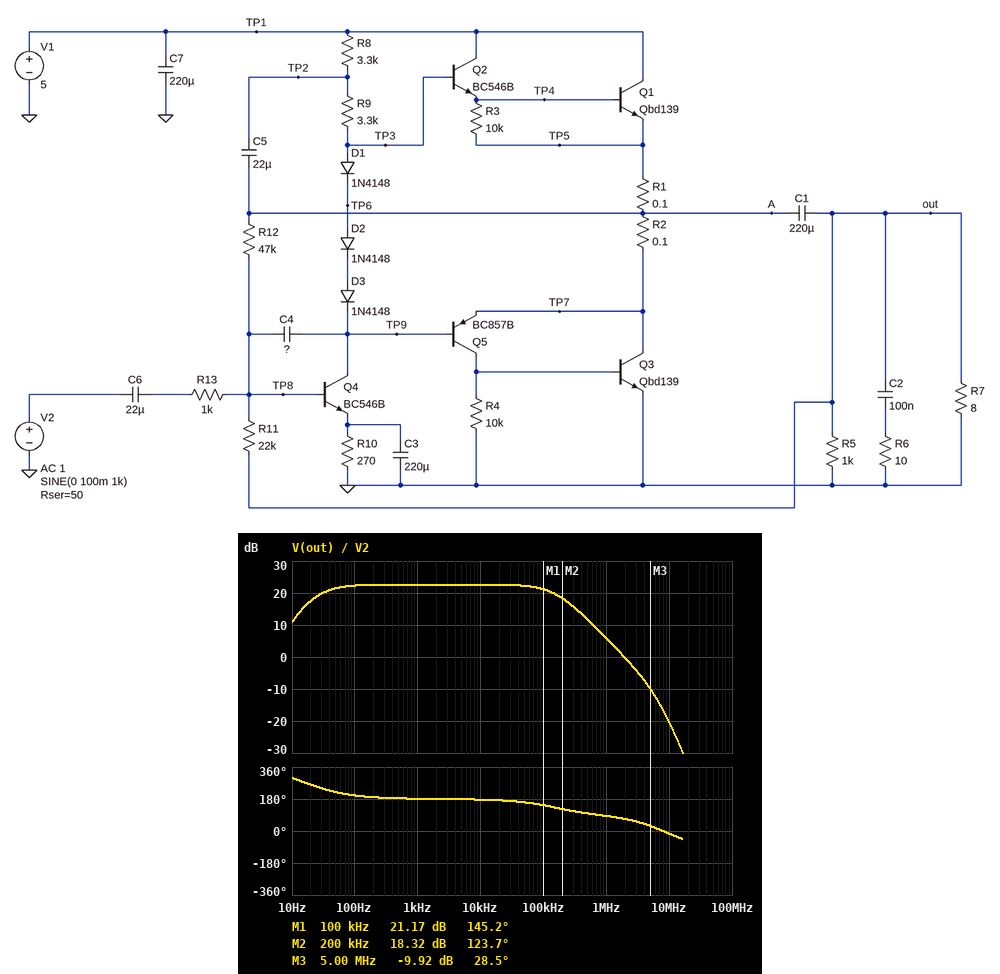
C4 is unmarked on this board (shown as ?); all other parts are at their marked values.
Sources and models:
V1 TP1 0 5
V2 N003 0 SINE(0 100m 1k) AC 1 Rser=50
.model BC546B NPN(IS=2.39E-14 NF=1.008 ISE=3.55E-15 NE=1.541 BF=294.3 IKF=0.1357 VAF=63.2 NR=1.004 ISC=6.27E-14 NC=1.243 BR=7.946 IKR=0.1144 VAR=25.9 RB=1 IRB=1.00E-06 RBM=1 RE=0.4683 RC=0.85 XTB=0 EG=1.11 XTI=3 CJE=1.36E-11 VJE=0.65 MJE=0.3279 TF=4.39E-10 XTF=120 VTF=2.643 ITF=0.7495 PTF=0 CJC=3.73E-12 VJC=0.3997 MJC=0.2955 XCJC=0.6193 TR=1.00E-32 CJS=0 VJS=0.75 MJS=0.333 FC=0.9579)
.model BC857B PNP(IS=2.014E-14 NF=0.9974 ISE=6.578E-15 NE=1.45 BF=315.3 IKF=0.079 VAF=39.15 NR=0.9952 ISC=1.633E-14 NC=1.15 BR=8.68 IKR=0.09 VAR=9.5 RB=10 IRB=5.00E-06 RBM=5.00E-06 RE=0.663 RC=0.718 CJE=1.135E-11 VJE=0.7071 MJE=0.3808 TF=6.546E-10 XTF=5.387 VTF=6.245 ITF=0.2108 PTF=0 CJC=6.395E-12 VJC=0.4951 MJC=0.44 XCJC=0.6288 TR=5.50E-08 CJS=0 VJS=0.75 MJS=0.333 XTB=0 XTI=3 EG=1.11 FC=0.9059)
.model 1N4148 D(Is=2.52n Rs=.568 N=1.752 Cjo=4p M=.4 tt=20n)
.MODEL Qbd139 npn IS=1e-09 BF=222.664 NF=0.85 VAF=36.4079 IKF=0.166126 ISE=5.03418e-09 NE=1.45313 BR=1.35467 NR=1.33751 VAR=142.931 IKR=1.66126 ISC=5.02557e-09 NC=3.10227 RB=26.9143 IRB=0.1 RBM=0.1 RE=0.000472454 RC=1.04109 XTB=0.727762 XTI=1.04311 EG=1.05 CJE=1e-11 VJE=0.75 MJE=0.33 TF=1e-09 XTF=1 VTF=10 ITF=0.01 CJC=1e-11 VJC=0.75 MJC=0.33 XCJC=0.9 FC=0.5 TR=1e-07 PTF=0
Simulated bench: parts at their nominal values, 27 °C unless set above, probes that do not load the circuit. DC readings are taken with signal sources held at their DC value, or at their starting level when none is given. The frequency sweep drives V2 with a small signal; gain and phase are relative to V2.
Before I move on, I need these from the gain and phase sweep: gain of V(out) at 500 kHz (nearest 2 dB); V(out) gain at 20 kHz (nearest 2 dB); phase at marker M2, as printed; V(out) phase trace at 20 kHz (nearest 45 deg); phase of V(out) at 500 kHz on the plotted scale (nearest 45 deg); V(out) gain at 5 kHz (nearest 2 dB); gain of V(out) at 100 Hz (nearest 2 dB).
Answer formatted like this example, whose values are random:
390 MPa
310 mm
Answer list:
12 dB
22 dB
123.7 deg
180 deg
90 deg
22 dB
22 dB
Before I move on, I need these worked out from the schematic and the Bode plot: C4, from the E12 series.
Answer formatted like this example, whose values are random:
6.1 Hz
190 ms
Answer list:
56 pF
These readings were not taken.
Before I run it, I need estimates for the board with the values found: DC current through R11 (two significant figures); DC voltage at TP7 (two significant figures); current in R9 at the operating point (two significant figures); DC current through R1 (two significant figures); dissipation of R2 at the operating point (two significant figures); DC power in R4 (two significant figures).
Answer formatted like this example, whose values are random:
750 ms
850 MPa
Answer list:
31 µA
2.2 V
280 µA
21 mA
43 µW
14 µW
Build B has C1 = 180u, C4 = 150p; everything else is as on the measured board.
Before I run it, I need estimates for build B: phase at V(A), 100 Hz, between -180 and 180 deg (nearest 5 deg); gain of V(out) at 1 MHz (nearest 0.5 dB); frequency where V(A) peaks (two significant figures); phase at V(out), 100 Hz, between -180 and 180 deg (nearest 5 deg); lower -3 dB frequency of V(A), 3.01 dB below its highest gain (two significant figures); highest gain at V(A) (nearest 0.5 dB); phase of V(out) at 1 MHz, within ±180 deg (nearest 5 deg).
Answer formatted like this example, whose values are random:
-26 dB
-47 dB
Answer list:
155 deg
-2.5 dB
18 Hz
-155 deg
7.4 Hz
31.5 dB
75 deg
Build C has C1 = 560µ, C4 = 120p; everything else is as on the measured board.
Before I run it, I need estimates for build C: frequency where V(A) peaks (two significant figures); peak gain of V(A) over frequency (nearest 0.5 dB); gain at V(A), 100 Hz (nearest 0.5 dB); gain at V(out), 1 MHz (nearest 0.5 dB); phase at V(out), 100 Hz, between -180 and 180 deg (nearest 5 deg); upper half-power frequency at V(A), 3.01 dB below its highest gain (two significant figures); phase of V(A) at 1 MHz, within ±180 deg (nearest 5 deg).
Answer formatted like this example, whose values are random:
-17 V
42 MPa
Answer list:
11 Hz
29.0 dB
23.0 dB
-0.5 dB
-170 deg
30 Hz
80 deg
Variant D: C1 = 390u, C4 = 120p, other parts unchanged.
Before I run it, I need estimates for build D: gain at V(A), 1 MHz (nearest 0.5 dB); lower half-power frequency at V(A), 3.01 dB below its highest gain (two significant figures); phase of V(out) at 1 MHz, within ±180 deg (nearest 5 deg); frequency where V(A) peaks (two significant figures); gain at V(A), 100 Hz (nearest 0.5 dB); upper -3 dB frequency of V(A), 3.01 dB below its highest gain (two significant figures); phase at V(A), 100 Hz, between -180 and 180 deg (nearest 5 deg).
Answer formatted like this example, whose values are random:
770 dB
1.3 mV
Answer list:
-0.5 dB
6.1 Hz
80 deg
13 Hz
23.5 dB
34 Hz
165 deg
